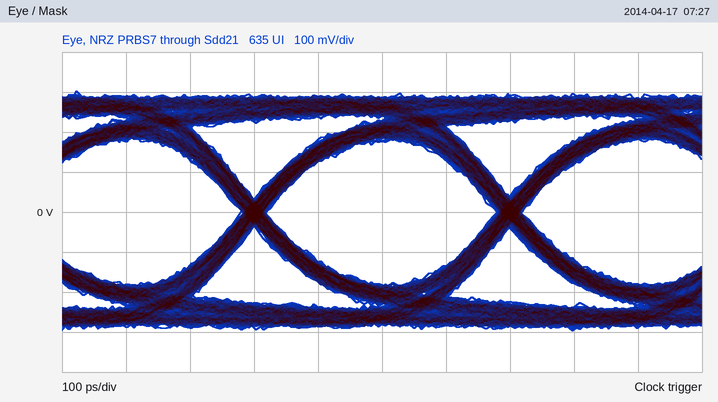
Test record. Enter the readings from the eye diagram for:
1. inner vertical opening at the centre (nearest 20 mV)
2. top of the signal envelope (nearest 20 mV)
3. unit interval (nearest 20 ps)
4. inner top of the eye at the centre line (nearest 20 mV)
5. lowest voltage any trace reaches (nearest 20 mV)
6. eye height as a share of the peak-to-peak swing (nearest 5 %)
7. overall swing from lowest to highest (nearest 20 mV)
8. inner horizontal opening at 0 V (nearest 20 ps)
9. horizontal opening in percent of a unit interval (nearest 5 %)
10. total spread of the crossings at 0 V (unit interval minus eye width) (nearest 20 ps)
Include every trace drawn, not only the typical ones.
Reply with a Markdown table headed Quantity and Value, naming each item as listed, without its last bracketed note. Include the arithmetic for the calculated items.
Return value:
| Quantity | Value |
|---|---|
| inner vertical opening at the centre | 360 mV |
| top of the signal envelope | 300 mV |
| unit interval | 400 ps |
| inner top of the eye at the centre line | 180 mV |
| lowest voltage any trace reaches | -300 mV |
| eye height as a share of the peak-to-peak swing | 360 mV / 600 mV ≈ 60 % |
| overall swing from lowest to highest | 600 mV |
| inner horizontal opening at 0 V | 360 ps |
| horizontal opening in percent of a unit interval | 360 ps / 400 ps ≈ 90 % |
| total spread of the crossings at 0 V (unit interval minus eye width) | 40 ps |
